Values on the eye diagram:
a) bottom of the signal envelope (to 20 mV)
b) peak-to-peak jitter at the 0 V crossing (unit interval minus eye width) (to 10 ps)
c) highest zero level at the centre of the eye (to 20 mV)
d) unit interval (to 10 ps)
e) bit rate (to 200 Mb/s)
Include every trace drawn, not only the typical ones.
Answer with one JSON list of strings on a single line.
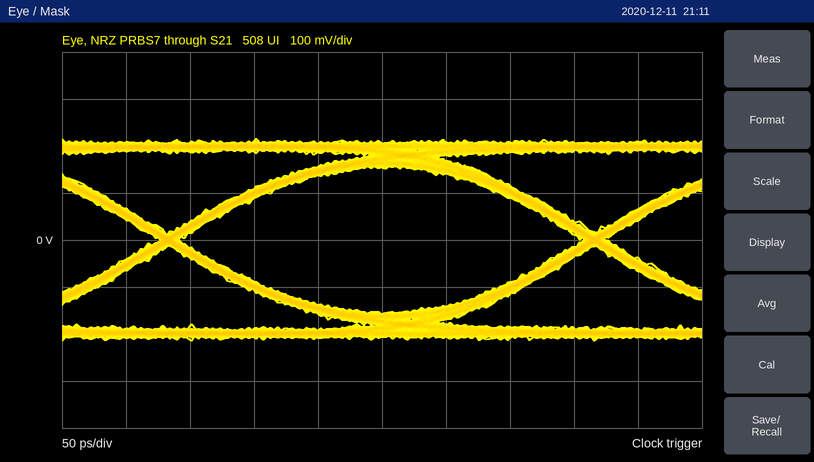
["-220 mV", "20 ps", "-160 mV", "330 ps", "3.0 Gb/s"]
